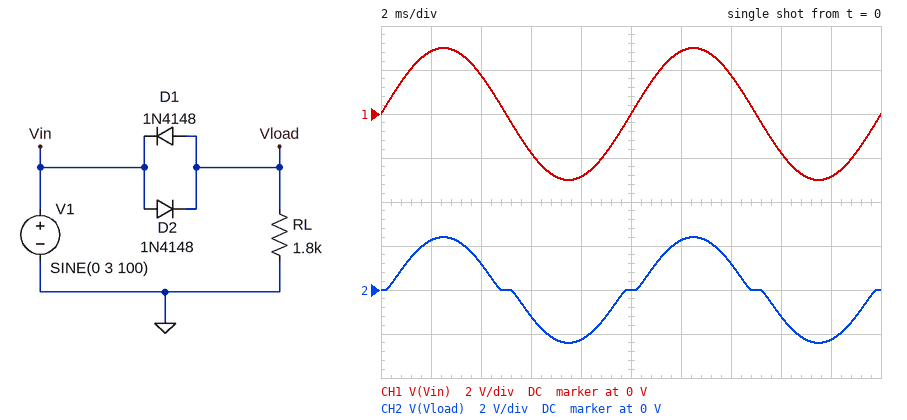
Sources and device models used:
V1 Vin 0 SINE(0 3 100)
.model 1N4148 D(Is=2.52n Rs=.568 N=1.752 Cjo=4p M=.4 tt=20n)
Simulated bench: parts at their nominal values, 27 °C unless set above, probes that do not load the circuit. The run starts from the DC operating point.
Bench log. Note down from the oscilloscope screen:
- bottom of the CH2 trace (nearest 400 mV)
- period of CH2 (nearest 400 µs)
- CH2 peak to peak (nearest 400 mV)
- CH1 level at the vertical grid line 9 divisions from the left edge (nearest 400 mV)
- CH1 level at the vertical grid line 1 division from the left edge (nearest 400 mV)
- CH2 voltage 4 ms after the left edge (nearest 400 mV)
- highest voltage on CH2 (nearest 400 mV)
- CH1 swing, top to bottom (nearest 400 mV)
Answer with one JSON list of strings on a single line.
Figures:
["-2.4 V", "10.0 ms", "4.8 V", "-2.8 V", "2.8 V", "1.2 V", "2.4 V", "6.0 V"]
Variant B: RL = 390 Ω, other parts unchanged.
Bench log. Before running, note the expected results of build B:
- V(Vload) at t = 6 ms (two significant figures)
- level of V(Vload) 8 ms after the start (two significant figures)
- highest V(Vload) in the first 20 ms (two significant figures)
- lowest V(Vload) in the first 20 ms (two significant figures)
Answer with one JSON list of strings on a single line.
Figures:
["-1.1 V", "-2.2 V", "2.3 V", "-2.3 V"]
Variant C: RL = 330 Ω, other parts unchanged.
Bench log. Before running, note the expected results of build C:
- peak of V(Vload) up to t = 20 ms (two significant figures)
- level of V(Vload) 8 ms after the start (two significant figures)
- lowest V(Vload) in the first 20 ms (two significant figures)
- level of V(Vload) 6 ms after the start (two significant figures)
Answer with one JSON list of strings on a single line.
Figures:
["2.3 V", "-2.2 V", "-2.3 V", "-1.1 V"]
